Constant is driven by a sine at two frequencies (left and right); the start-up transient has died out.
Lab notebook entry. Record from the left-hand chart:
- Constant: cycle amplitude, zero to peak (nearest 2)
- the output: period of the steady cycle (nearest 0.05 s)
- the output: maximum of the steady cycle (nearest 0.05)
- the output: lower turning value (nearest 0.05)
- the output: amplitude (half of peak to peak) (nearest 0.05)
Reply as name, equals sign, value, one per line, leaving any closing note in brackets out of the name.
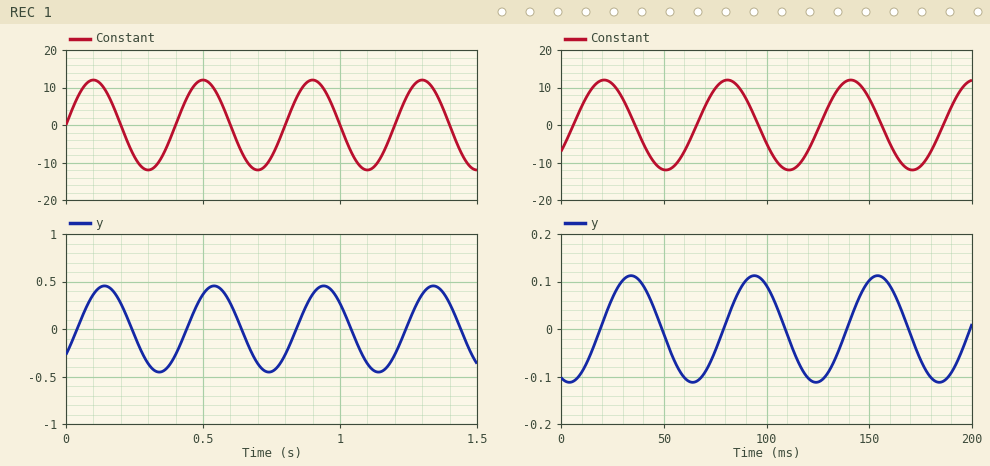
Constant: cycle amplitude, zero to peak = 12
the output: period of the steady cycle = 0.40 s
the output: maximum of the steady cycle = 0.45
the output: lower turning value = -0.45
the output: amplitude (half of peak to peak) = 0.45
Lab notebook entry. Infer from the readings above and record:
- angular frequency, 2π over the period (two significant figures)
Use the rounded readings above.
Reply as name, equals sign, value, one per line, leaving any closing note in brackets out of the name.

angular frequency, 2π over the period = 16 rad/s
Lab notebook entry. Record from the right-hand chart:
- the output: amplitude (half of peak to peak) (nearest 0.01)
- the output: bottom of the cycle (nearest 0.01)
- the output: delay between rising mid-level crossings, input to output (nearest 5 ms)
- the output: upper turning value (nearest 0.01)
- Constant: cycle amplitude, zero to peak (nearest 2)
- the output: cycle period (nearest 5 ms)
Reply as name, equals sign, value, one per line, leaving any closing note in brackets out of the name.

the output: amplitude (half of peak to peak) = 0.11
the output: bottom of the cycle = -0.11
the output: delay between rising mid-level crossings, input to output = 15 ms
the output: upper turning value = 0.11
Constant: cycle amplitude, zero to peak = 12
the output: cycle period = 60 ms
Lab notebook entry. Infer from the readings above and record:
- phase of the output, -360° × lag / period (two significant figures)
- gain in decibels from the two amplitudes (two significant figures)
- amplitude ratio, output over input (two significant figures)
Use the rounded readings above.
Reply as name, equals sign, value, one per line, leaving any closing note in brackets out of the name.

phase of the output, -360° × lag / period = -90°
gain in decibels from the two amplitudes = -41 dB
amplitude ratio, output over input = 0.0092
